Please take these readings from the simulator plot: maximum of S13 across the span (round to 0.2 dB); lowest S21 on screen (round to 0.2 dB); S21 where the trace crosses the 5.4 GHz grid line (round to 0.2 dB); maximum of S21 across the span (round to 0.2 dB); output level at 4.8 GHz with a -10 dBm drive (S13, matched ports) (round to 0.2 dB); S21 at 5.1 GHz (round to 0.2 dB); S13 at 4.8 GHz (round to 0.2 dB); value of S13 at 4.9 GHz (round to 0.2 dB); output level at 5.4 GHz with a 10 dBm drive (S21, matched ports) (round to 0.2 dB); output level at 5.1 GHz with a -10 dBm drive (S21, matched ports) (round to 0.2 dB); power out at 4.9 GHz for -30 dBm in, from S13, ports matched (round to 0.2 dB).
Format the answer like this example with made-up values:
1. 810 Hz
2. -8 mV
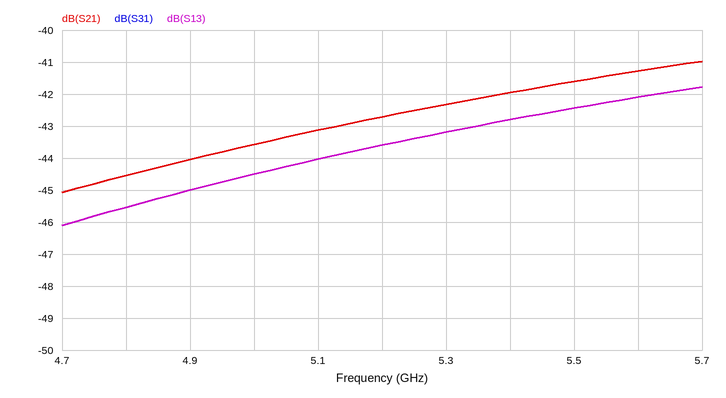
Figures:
1. -41.8 dB
2. -45.0 dB
3. -42.0 dB
4. -41.0 dB
5. -55.6 dBm
6. -43.2 dB
7. -45.6 dB
8. -45.0 dB
9. -32.0 dBm
10. -53.2 dBm
11. -75.0 dBm
